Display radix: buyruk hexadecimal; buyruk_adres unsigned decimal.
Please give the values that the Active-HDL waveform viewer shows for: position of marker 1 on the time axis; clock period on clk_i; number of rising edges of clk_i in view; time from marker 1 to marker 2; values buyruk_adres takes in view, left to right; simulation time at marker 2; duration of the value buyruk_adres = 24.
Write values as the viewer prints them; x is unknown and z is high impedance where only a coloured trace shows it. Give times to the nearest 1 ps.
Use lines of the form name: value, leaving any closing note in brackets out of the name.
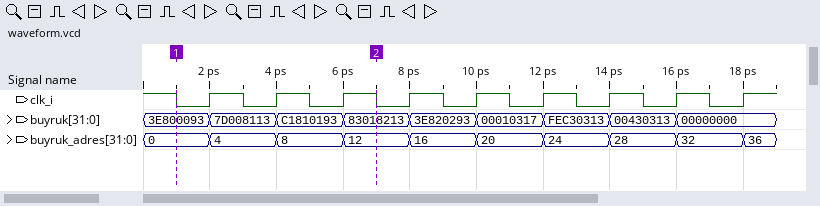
position of marker 1 on the time axis: 1 ps
clock period on clk_i: 2 ps
number of rising edges of clk_i in view: 9
time from marker 1 to marker 2: 6 ps
values buyruk_adres takes in view, left to right: 0, 4, 8, 12, 16, 20, 24, 28, 32, 36
simulation time at marker 2: 7 ps
duration of the value buyruk_adres = 24: 2 ps
